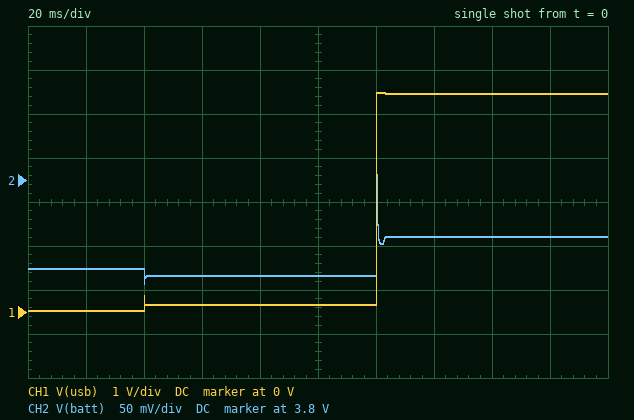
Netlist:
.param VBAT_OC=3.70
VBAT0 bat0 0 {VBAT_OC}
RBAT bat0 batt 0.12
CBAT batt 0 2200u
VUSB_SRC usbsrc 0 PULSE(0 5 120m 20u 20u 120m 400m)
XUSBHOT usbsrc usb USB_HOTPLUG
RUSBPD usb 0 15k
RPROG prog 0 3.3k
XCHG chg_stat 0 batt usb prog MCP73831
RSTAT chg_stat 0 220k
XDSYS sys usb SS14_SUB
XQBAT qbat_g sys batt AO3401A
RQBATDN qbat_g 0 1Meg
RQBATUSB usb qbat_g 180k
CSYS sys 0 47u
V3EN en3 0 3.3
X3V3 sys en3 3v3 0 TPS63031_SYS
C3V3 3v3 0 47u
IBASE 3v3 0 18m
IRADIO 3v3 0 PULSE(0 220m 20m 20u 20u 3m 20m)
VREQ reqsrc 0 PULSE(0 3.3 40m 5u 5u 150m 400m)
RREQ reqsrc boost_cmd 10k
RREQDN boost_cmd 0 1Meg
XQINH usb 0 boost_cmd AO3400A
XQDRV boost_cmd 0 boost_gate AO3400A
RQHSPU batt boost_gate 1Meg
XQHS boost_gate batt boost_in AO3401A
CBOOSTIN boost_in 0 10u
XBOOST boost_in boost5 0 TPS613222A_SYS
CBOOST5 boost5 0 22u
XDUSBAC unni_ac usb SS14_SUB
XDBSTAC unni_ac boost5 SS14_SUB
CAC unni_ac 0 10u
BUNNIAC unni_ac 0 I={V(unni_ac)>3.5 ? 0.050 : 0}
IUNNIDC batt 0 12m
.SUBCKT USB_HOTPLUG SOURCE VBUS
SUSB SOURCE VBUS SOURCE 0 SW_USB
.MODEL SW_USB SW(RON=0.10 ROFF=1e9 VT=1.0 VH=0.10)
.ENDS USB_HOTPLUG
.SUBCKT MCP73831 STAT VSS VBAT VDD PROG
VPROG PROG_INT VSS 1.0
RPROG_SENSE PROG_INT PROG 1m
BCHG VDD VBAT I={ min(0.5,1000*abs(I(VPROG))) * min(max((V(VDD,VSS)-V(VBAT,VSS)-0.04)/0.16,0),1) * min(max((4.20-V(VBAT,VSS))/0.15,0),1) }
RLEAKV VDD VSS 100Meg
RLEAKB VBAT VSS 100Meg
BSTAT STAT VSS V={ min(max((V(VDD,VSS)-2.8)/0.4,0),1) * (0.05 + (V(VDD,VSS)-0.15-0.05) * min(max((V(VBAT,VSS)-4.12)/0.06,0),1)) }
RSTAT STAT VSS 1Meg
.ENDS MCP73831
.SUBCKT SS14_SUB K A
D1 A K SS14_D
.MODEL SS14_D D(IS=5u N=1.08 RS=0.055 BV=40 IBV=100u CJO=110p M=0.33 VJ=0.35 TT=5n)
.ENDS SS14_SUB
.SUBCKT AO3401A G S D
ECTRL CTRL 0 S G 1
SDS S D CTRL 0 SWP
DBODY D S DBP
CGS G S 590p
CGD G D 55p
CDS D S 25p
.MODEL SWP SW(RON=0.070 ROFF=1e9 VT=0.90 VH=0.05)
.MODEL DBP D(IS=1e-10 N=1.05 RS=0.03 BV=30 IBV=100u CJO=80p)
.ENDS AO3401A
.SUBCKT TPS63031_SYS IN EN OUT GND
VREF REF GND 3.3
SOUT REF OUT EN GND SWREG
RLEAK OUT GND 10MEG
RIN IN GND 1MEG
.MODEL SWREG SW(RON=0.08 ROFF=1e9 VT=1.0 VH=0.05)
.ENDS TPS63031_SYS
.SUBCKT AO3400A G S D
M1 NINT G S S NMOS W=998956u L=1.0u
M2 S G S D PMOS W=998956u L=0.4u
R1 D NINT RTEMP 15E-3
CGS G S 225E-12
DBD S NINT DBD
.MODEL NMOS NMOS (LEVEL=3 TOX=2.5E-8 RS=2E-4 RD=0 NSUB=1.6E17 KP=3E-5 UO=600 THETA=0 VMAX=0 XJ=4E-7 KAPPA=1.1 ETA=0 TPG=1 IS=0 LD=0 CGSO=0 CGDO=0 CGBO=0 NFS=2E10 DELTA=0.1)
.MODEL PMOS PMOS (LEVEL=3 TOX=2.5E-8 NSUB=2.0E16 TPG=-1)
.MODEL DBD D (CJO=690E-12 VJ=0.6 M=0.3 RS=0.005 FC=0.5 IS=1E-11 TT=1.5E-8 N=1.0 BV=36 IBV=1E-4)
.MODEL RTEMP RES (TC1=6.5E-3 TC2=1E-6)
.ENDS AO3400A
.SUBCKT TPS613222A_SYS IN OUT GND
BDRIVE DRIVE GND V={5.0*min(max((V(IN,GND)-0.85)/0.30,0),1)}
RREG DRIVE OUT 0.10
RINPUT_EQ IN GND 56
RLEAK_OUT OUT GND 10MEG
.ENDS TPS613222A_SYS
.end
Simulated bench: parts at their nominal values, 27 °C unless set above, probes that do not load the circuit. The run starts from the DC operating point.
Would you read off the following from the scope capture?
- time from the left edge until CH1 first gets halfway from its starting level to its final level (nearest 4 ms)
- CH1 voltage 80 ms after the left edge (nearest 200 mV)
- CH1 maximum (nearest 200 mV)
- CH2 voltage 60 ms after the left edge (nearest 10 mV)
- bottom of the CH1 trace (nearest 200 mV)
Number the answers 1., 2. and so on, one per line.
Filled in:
1. 120 ms
2. 200 mV
3. 5.0 V
4. 3.69 V
5. 0 V
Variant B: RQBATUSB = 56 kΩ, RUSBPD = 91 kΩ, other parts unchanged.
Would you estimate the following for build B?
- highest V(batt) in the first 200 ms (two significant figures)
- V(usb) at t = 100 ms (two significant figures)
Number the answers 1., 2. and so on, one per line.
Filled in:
1. 3.7 V
2. 840 mV
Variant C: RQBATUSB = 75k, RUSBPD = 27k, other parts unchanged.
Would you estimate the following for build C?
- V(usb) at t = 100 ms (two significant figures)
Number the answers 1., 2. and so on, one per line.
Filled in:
1. 260 mV
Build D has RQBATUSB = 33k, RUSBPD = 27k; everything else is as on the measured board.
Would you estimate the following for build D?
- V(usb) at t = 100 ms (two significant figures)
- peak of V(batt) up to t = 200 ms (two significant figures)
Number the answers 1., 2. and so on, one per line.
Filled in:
1. 260 mV
2. 3.7 V
